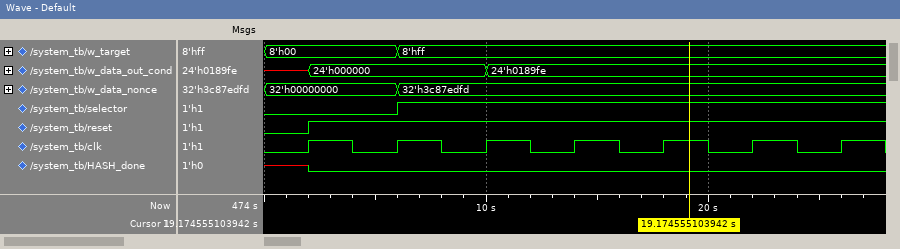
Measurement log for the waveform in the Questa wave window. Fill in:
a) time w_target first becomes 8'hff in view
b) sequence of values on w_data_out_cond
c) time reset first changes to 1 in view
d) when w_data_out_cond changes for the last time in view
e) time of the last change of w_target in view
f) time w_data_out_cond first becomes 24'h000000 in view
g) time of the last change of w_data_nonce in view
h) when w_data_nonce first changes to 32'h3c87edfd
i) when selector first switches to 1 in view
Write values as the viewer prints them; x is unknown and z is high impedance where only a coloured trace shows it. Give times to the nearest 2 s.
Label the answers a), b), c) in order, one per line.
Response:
a) 6 s
b) x, 24'h000000, 24'h0189fe
c) 2 s
d) 10 s
e) 6 s
f) 2 s
g) 6 s
h) 6 s
i) 6 s
